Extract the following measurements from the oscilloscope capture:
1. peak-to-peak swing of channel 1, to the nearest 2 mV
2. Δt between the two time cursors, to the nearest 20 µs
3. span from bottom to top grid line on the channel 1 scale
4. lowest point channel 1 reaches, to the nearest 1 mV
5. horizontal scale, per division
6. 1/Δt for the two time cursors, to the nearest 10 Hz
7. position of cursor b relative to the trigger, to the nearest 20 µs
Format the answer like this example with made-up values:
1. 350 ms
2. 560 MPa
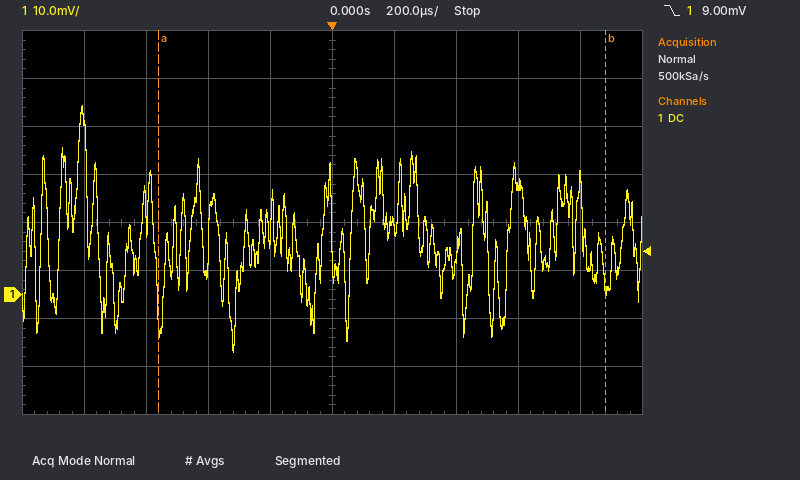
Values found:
1. 52 mV
2. 1.44 ms
3. 80 mV
4. -12 mV
5. 200 µs
6. 690 Hz
7. +880 µs
